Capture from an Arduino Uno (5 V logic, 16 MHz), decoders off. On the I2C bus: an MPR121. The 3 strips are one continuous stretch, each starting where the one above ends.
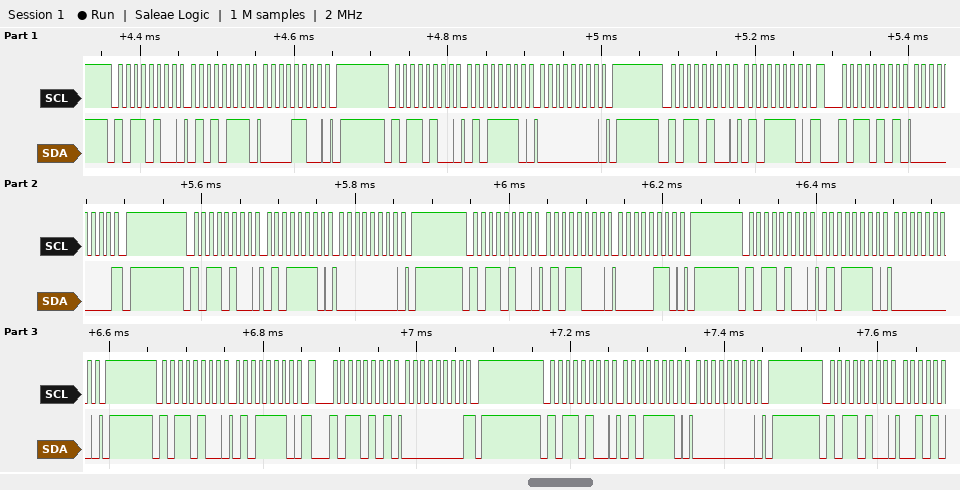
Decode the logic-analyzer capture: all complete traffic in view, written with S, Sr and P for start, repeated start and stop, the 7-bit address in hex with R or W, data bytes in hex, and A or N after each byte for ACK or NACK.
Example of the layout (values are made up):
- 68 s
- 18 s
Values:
- S 5AW A 57 A 0C A P S 5AW A 5E A 00 A P S 5AW A 5E A Sr 5AR A 00 N P S 5AW A 5E A 00 A P S 5AW A 58 A 06 A P S 5AW A 5E A 00 A P S 5AW A 5E A Sr 5AR A 00 N P S 5AW A 5E A 00 A P S 5AW A
